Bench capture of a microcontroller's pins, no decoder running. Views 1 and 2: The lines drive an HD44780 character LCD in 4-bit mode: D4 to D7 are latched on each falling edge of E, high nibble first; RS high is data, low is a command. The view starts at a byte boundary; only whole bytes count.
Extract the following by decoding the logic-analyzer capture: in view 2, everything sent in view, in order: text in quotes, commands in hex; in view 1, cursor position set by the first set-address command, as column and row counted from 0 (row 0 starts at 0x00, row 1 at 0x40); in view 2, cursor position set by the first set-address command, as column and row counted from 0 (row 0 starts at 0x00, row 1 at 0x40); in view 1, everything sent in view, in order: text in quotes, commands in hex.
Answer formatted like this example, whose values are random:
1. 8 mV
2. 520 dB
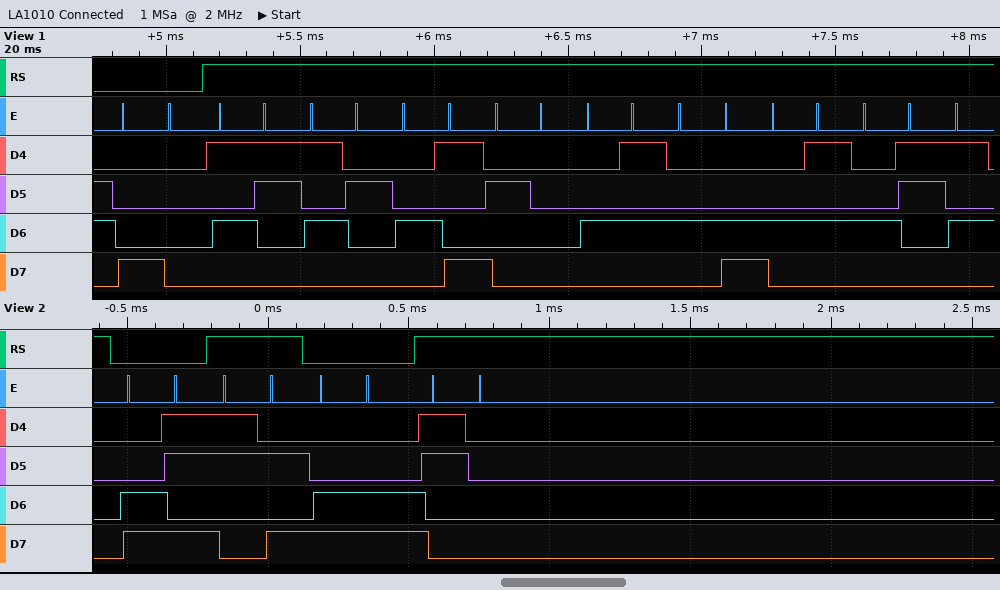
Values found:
1. 0xCB ":" 0xCC "0"
2. column 0, row 0
3. column 11, row 1
4. 0x80 "SRI ELEC"
